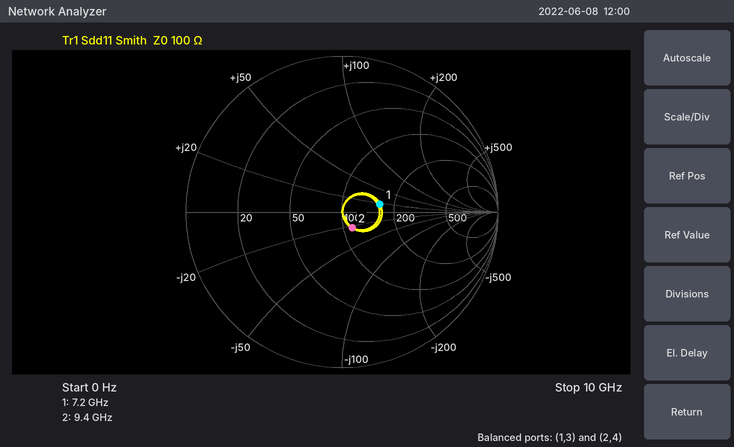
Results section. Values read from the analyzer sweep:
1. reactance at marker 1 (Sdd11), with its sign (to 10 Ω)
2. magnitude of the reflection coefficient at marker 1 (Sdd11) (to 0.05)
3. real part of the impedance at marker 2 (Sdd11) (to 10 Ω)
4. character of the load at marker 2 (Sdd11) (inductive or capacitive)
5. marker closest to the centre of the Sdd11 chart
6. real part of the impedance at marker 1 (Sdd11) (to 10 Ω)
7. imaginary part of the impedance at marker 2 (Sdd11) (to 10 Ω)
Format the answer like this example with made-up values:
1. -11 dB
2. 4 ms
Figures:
1. +20 Ω
2. 0.25
3. 110 Ω
4. capacitive
5. marker 2
6. 160 Ω
7. -20 Ω
